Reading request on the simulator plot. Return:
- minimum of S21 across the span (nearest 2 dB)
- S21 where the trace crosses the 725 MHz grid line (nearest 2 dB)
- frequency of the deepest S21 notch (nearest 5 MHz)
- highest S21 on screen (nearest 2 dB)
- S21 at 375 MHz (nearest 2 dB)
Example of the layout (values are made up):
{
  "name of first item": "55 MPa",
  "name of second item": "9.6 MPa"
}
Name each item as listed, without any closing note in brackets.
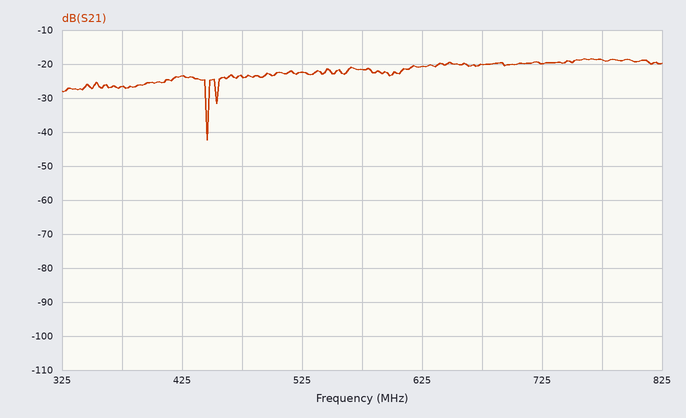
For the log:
{
  "minimum of S21 across the span": "-42 dB",
  "S21 where the trace crosses the 725 MHz grid line": "-20 dB",
  "frequency of the deepest S21 notch": "445 MHz",
  "highest S21 on screen": "-18 dB",
  "S21 at 375 MHz": "-26 dB"
}
